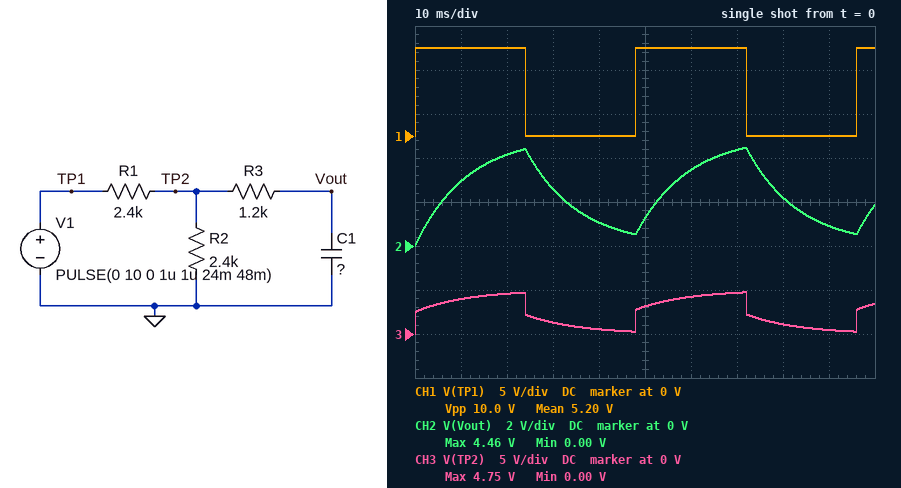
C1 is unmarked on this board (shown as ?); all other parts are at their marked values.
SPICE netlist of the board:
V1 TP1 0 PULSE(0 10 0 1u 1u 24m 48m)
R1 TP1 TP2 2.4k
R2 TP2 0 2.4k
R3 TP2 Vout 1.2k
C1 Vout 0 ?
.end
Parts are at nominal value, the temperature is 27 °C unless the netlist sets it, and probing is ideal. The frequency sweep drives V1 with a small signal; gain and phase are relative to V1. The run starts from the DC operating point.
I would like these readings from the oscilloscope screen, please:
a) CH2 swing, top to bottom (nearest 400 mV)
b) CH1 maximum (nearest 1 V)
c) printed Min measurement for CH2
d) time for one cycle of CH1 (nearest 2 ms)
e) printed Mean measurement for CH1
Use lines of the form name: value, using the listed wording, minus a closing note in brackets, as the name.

CH2 swing, top to bottom: 4.4 V
CH1 maximum: 10 V
printed Min measurement for CH2: 0.00 V
time for one cycle of CH1: 48 ms
printed Mean measurement for CH1: 5.20 V
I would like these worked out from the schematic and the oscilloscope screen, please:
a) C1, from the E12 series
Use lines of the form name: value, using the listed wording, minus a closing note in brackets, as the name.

C1, from the E12 series: 4.7 µF
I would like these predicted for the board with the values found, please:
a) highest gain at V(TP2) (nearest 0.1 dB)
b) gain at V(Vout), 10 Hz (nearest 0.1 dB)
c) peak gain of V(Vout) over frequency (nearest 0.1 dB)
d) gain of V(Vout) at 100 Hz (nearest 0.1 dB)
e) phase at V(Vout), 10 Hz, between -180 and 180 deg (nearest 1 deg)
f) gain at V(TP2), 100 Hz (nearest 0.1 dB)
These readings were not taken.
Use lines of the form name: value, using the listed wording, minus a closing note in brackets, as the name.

highest gain at V(TP2): -6.0 dB
gain at V(Vout), 10 Hz: -7.8 dB
peak gain of V(Vout) over frequency: -6.0 dB
gain of V(Vout) at 100 Hz: -23.1 dB
phase at V(Vout), 10 Hz, between -180 and 180 deg: -35 deg
gain at V(TP2), 100 Hz: -11.8 dB
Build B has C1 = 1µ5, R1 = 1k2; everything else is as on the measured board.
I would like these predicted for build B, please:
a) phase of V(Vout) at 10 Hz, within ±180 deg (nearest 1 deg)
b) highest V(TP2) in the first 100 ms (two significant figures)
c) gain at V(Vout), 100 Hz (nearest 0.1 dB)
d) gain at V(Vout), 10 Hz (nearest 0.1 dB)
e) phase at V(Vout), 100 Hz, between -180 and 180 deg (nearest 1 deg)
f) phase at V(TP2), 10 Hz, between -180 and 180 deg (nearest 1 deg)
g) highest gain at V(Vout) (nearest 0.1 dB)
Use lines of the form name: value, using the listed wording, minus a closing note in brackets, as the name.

phase of V(Vout) at 10 Hz, within ±180 deg: -11 deg
highest V(TP2) in the first 100 ms: 6.7 V
gain at V(Vout), 100 Hz: -10.1 dB
gain at V(Vout), 10 Hz: -3.7 dB
phase at V(Vout), 100 Hz, between -180 and 180 deg: -62 deg
phase at V(TP2), 10 Hz, between -180 and 180 deg: -4 deg
highest gain at V(Vout): -3.5 dB
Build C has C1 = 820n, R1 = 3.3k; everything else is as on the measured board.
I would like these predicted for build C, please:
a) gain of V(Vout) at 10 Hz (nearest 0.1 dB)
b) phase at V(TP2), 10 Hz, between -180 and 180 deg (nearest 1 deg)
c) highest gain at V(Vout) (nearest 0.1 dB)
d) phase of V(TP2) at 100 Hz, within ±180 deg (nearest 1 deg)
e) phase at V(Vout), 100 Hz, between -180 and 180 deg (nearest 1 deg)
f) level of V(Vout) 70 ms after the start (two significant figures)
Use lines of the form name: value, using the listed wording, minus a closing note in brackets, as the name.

gain of V(Vout) at 10 Hz: -7.6 dB
phase at V(TP2), 10 Hz, between -180 and 180 deg: -4 deg
highest gain at V(Vout): -7.5 dB
phase of V(TP2) at 100 Hz, within ±180 deg: -21 deg
phase at V(Vout), 100 Hz, between -180 and 180 deg: -53 deg
level of V(Vout) 70 ms after the start: 4.2 V
